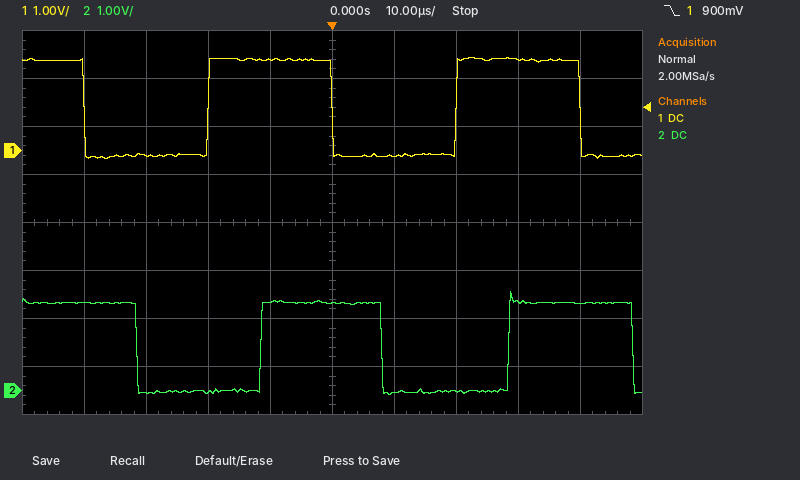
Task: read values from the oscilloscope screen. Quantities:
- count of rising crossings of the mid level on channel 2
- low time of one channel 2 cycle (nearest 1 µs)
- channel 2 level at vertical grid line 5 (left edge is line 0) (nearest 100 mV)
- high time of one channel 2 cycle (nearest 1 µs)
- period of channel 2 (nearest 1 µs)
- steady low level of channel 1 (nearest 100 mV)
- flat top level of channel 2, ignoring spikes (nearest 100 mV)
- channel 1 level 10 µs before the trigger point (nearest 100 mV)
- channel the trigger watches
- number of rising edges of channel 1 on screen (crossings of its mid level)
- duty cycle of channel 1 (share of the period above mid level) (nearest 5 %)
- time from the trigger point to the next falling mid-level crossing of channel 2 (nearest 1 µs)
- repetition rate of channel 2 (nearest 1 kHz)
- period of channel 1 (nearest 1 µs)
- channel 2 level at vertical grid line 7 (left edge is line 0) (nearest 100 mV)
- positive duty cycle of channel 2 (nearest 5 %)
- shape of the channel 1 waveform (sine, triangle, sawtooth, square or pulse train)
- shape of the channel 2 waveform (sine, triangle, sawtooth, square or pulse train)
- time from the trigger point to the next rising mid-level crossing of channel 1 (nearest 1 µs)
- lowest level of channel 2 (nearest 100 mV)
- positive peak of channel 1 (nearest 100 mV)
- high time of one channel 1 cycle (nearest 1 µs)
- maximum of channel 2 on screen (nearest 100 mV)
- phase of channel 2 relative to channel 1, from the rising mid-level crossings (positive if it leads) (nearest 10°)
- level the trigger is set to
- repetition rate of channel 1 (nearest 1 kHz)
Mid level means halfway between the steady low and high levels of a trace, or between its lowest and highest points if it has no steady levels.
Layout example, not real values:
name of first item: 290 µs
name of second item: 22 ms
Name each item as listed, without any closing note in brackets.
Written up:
count of rising crossings of the mid level on channel 2: 2
low time of one channel 2 cycle: 20 µs
channel 2 level at vertical grid line 5 (left edge is line 0): 1.8 V
high time of one channel 2 cycle: 20 µs
period of channel 2: 40 µs
steady low level of channel 1: -100 mV
flat top level of channel 2, ignoring spikes: 1.8 V
channel 1 level 10 µs before the trigger point: 1.9 V
channel the trigger watches: channel 1
number of rising edges of channel 1 on screen: 2
duty cycle of channel 1 (share of the period above mid level): 50 %
time from the trigger point to the next falling mid-level crossing of channel 2: 8 µs
repetition rate of channel 2: 25 kHz
period of channel 1: 40 µs
channel 2 level at vertical grid line 7 (left edge is line 0): 0.0 V
positive duty cycle of channel 2: 50 %
shape of the channel 1 waveform: square
shape of the channel 2 waveform: square
time from the trigger point to the next rising mid-level crossing of channel 1: 20 µs
lowest level of channel 2: -100 mV
positive peak of channel 1: 1.9 V
high time of one channel 1 cycle: 20 µs
maximum of channel 2 on screen: 2.1 V
phase of channel 2 relative to channel 1, from the rising mid-level crossings (positive if it leads): -80°
level the trigger is set to: 900 mV
repetition rate of channel 1: 25 kHz
